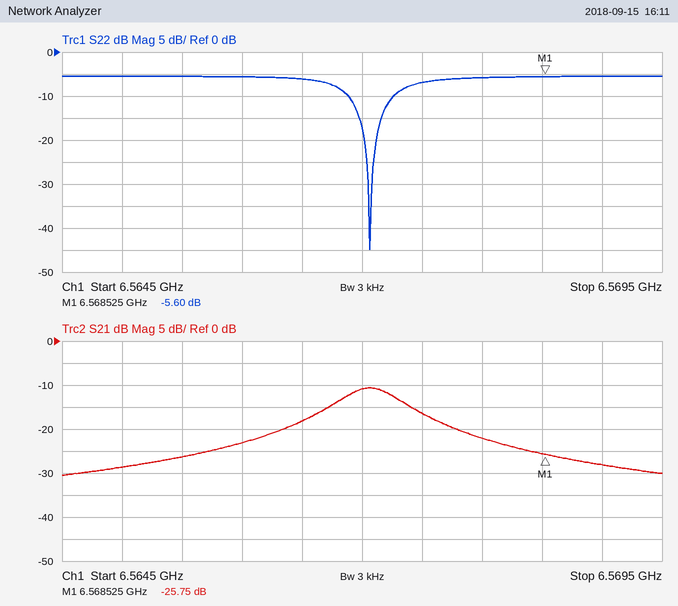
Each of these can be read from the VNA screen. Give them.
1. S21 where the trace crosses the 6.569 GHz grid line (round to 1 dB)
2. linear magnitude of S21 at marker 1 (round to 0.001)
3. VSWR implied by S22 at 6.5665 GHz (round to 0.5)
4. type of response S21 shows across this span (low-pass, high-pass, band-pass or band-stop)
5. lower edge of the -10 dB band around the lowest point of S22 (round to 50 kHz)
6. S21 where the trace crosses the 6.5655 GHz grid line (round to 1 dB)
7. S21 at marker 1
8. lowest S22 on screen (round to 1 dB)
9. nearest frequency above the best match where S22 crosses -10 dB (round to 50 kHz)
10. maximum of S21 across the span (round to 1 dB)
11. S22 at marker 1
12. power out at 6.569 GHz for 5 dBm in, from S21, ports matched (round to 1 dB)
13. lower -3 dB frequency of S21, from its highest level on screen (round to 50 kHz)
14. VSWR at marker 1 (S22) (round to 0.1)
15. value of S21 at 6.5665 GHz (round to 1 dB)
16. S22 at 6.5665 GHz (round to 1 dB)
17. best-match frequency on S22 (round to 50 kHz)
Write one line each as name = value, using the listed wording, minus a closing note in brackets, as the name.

S21 where the trace crosses the 6.569 GHz grid line = -28 dB
linear magnitude of S21 at marker 1 = 0.052
VSWR implied by S22 at 6.5665 GHz = 3.0
type of response S21 shows across this span = band-pass
lower edge of the -10 dB band around the lowest point of S22 = 6.56690 GHz
S21 where the trace crosses the 6.5655 GHz grid line = -26 dB
S21 at marker 1 = -25.75 dB
lowest S22 on screen = -45 dB
nearest frequency above the best match where S22 crosses -10 dB = 6.56725 GHz
maximum of S21 across the span = -11 dB
S22 at marker 1 = -5.60 dB
power out at 6.569 GHz for 5 dBm in, from S21, ports matched = -23 dBm
lower -3 dB frequency of S21, from its highest level on screen = 6.56680 GHz
VSWR at marker 1 (S22) = 3.2
value of S21 at 6.5665 GHz = -18 dB
S22 at 6.5665 GHz = -6 dB
best-match frequency on S22 = 6.56705 GHz
